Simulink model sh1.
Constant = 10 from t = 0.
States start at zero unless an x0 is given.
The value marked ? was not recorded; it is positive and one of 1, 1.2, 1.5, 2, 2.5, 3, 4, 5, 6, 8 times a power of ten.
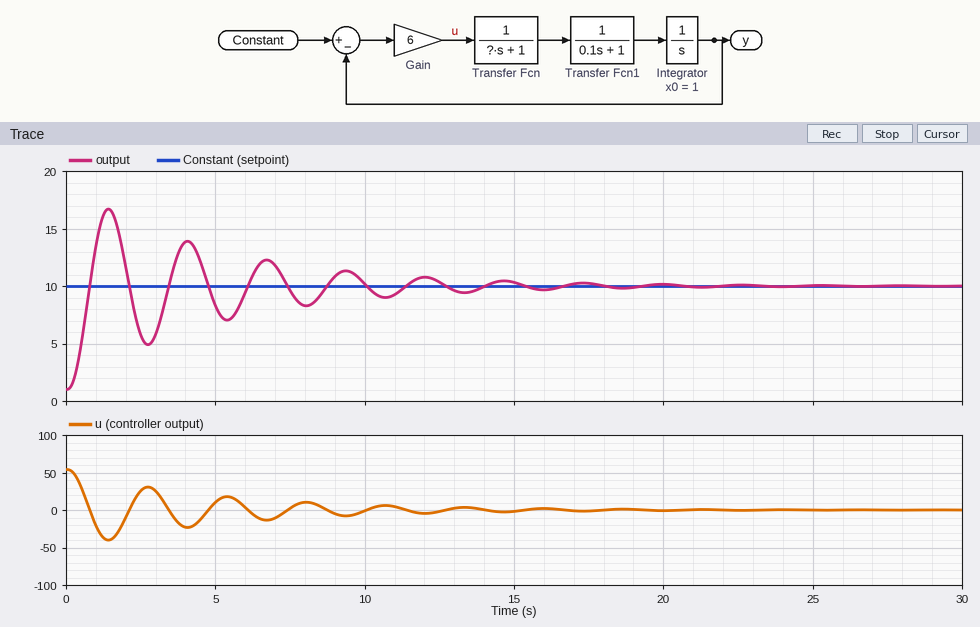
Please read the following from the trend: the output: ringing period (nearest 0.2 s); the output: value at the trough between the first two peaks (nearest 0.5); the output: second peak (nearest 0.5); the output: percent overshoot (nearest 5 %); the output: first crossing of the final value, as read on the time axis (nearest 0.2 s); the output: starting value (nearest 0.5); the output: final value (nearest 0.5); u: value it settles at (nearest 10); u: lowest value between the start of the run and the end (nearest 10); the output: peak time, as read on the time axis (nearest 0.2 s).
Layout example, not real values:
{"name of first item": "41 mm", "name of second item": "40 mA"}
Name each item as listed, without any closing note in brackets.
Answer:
{"the output: ringing period": "2.6 s", "the output: value at the trough between the first two peaks": "5.0", "the output: second peak": "14.0", "the output: percent overshoot": "75 %", "the output: first crossing of the final value, as read on the time axis": "0.8 s", "the output: starting value": "1.0", "the output: final value": "10.0", "u: value it settles at": "0", "u: lowest value between the start of the run and the end": "-40", "the output: peak time, as read on the time axis": "1.4 s"}
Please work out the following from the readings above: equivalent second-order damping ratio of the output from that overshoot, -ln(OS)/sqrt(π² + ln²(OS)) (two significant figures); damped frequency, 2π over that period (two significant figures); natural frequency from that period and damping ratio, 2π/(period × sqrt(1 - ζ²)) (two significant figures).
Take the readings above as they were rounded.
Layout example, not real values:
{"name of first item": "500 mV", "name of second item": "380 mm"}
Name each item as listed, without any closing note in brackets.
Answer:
{"equivalent second-order damping ratio of the output from that overshoot, -ln(OS)/sqrt(π² + ln²(OS))": "0.091", "damped frequency, 2π over that period": "2.4 rad/s", "natural frequency from that period and damping ratio, 2π/(period × sqrt(1 - ζ²))": "2.4 rad/s"}
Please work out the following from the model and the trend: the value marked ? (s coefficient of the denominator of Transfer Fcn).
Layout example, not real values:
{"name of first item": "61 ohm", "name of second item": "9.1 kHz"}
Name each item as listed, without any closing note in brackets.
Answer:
{"the value marked ?": "1"}
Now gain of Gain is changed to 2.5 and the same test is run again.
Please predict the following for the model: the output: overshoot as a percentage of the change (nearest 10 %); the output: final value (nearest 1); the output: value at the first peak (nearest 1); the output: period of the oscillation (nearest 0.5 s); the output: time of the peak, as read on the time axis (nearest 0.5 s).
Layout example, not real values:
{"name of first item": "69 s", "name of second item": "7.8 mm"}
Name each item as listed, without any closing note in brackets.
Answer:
{"the output: overshoot as a percentage of the change": "50 %", "the output: final value": "10", "the output: value at the first peak": "14", "the output: period of the oscillation": "4.0 s", "the output: time of the peak, as read on the time axis": "2.0 s"}
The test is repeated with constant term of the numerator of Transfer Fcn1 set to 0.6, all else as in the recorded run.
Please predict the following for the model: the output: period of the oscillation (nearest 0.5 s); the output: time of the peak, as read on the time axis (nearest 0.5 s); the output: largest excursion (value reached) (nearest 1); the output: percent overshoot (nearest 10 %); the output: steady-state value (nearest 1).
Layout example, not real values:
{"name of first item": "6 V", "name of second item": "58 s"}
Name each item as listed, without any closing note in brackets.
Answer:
{"the output: period of the oscillation": "3.5 s", "the output: time of the peak, as read on the time axis": "2.0 s", "the output: largest excursion (value reached)": "15", "the output: percent overshoot": "60 %", "the output: steady-state value": "10"}
